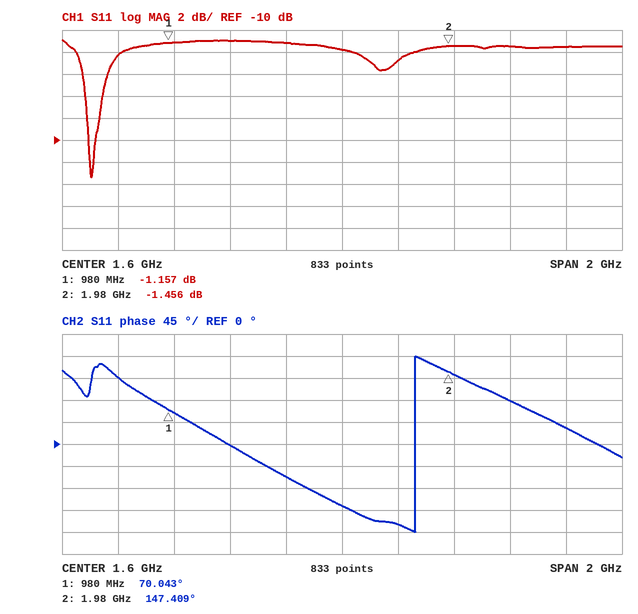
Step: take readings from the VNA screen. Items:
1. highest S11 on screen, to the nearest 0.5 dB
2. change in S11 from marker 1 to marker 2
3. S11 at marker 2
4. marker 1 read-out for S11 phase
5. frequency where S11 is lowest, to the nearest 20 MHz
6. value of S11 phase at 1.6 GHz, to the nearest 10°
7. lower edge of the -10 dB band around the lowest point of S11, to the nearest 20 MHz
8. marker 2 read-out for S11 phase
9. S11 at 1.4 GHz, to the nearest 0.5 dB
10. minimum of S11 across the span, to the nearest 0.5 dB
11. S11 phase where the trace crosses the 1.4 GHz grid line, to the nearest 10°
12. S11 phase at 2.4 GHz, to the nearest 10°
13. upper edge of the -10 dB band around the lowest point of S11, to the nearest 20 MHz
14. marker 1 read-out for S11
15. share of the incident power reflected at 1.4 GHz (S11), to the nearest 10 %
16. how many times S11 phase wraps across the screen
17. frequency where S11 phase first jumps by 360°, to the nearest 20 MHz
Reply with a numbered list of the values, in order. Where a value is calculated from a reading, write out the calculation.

1. -1.0 dB
2. -1.456 − (-1.157) = -0.299 dB
3. -1.456 dB
4. 70.043°
5. 700 MHz
6. -130°
7. 700 MHz
8. 147.409°
9. -1.0 dB
10. -13.5 dB
11. -70°
12. 30°
13. 720 MHz
14. -1.157 dB
15. 10^(-1/10) ≈ 79.4 %, so 80 % to the nearest 10 %
16. 1
17. 1.86 GHz
